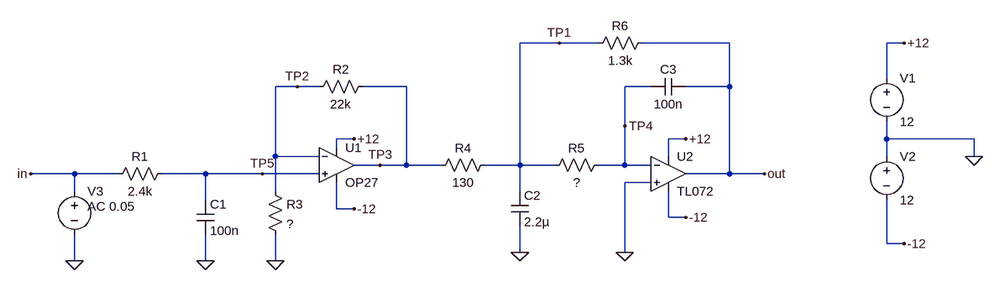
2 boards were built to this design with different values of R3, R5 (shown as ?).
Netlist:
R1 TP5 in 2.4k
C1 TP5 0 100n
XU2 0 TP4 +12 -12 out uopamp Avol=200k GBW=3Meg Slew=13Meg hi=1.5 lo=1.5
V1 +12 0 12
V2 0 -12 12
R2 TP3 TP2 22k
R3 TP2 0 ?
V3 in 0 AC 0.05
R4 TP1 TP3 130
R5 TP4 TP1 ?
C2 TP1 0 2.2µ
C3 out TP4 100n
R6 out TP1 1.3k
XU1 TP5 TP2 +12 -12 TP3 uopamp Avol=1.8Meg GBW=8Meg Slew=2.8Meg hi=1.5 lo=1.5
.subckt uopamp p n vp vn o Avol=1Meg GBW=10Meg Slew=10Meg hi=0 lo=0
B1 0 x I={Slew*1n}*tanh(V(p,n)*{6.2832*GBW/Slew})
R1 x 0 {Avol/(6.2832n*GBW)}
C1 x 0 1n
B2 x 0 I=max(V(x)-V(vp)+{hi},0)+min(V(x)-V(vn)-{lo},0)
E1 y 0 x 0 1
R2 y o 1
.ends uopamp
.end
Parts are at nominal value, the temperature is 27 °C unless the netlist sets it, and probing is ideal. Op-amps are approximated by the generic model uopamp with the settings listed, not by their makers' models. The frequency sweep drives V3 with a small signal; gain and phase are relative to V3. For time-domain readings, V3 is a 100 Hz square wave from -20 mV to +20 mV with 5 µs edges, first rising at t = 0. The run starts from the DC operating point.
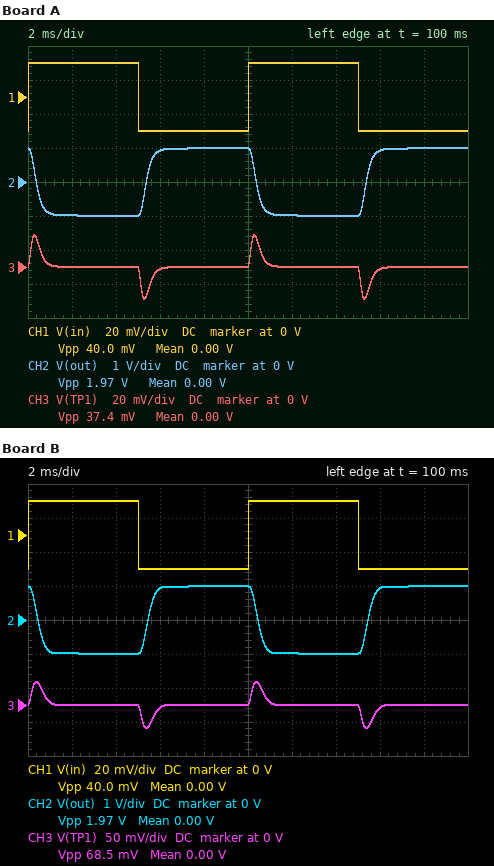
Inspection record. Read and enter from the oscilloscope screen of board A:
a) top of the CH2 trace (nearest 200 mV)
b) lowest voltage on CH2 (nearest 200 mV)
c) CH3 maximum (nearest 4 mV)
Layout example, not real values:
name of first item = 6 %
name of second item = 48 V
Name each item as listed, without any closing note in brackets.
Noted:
top of the CH2 trace = 1.0 V
lowest voltage on CH2 = -1.0 V
CH3 maximum = 20 mV
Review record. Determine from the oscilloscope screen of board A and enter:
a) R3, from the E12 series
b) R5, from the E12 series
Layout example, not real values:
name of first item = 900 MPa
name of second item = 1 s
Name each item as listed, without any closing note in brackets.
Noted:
R3, from the E12 series = 5.6 kΩ
R5, from the E12 series = 47 Ω
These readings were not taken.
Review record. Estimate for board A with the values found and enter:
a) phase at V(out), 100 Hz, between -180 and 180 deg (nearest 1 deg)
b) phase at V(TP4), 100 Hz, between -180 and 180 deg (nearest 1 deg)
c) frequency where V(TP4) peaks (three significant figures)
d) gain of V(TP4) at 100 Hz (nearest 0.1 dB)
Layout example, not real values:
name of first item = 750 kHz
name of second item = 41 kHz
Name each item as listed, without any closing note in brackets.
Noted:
phase at V(out), 100 Hz, between -180 and 180 deg = 165 deg
phase at V(TP4), 100 Hz, between -180 and 180 deg = 66 deg
frequency where V(TP4) peaks = 863 Hz
gain of V(TP4) at 100 Hz = -55.7 dB
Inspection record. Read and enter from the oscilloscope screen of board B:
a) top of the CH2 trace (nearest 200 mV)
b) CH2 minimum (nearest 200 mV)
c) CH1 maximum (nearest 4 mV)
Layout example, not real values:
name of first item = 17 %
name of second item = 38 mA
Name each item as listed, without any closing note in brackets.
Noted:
top of the CH2 trace = 1.0 V
CH2 minimum = -1.0 V
CH1 maximum = 20 mV
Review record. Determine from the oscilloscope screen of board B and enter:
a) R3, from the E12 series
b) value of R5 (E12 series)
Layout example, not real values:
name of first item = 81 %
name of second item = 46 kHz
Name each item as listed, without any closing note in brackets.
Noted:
R3, from the E12 series = 5.6 kΩ
value of R5 = 100 Ω
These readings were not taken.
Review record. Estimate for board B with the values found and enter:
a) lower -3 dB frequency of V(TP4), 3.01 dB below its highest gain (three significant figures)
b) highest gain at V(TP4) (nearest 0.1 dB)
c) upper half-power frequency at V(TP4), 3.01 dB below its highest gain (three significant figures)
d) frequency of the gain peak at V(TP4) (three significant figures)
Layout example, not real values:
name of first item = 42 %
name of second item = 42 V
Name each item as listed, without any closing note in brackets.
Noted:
lower -3 dB frequency of V(TP4), 3.01 dB below its highest gain = 335 Hz
highest gain at V(TP4) = -43.2 dB
upper half-power frequency at V(TP4), 3.01 dB below its highest gain = 1.22 kHz
frequency of the gain peak at V(TP4) = 699 Hz
